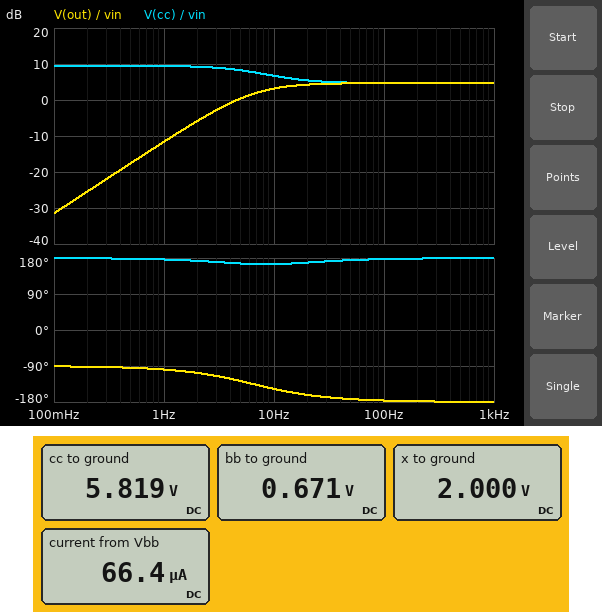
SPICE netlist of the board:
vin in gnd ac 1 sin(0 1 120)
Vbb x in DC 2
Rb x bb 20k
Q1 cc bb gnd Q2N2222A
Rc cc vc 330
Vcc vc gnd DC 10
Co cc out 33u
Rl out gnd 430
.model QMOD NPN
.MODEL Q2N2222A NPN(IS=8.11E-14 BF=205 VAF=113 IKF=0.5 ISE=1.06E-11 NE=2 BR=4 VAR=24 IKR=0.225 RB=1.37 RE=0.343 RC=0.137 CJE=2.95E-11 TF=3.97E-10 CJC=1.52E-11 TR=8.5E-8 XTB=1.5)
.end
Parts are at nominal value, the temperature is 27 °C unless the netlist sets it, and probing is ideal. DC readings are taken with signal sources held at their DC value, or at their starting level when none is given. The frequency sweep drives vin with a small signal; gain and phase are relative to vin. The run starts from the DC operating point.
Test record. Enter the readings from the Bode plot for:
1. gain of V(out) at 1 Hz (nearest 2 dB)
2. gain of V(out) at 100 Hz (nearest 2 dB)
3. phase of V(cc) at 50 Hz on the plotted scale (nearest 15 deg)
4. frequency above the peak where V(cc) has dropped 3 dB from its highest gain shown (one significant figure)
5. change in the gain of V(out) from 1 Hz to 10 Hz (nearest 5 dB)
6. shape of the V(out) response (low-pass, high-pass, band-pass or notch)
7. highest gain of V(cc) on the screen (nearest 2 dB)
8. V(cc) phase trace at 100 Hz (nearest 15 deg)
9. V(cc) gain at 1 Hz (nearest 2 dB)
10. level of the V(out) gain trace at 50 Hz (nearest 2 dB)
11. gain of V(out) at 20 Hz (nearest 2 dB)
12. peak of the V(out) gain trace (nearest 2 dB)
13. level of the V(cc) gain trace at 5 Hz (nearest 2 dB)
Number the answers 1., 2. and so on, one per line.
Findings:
1. -12 dB
2. 4 dB
3. 180 deg
4. 10 Hz
5. 15 dB
6. high-pass
7. 10 dB
8. 180 deg
9. 10 dB
10. 4 dB
11. 4 dB
12. 4 dB
13. 8 dB
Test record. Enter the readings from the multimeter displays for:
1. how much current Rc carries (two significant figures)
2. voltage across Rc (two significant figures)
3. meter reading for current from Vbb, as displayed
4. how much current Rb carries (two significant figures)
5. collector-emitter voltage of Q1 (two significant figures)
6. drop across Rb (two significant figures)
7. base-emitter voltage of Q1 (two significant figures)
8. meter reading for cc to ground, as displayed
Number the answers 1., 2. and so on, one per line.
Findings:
1. 13 mA
2. 4.2 V
3. 66.4 µA
4. 66 µA
5. 5.8 V
6. 1.3 V
7. 670 mV
8. 5.819 V
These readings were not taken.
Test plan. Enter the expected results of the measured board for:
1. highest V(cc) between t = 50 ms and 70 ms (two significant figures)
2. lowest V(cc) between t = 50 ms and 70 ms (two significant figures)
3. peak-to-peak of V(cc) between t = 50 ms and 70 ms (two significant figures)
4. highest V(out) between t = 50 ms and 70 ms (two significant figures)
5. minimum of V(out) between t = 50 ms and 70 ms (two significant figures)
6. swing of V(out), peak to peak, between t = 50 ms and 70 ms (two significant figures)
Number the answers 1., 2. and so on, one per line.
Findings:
1. 7.6 V
2. 4.1 V
3. 3.4 V
4. 1.7 V
5. -1.7 V
6. 3.4 V
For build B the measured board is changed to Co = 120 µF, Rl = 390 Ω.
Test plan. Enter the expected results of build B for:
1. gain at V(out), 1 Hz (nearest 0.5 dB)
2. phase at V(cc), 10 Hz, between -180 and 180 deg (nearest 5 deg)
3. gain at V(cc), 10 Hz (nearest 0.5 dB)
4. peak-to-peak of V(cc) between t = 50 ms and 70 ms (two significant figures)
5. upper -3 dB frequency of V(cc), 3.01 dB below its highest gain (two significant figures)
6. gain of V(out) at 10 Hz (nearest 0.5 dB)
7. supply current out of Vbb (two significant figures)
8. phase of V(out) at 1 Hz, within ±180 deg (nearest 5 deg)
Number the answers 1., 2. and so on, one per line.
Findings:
1. -2.0 dB
2. 170 deg
3. 4.5 dB
4. 3.3 V
5. 3.0 Hz
6. 4.0 dB
7. 66 µA
8. -120 deg
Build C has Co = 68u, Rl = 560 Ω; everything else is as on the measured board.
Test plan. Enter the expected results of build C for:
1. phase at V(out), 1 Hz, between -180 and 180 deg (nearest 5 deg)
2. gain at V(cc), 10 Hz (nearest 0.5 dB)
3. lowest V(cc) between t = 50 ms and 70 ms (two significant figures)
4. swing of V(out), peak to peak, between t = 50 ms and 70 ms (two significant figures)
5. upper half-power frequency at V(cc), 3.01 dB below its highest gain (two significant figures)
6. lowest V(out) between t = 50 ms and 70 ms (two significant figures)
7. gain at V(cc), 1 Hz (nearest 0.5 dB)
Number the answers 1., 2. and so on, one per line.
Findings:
1. -110 deg
2. 6.0 dB
3. 4.0 V
4. 3.8 V
5. 6.2 Hz
6. -1.9 V
7. 9.0 dB
